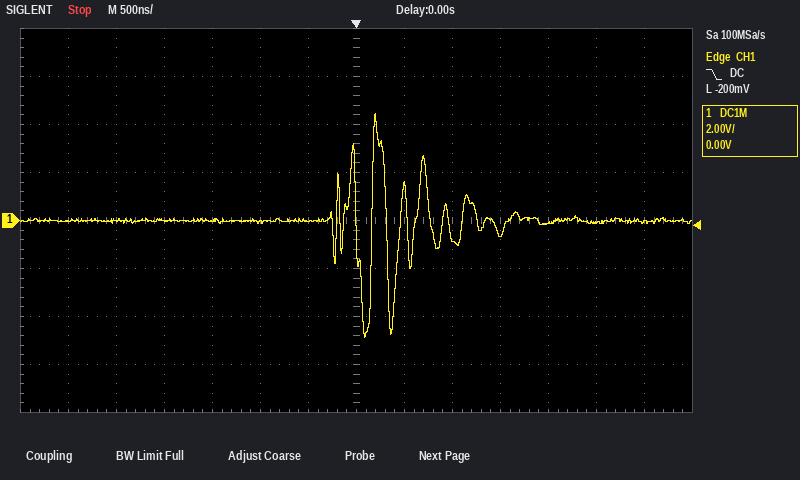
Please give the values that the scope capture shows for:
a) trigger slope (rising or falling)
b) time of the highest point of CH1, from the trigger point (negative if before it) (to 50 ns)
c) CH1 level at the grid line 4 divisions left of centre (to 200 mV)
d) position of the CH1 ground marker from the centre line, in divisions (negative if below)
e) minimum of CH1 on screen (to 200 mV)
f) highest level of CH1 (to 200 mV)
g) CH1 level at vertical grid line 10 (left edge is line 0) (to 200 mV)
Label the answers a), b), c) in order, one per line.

a) falling
b) +200 ns
c) 0.0 V
d) 0.0 div
e) -4.8 V
f) 4.4 V
g) -600 mV
